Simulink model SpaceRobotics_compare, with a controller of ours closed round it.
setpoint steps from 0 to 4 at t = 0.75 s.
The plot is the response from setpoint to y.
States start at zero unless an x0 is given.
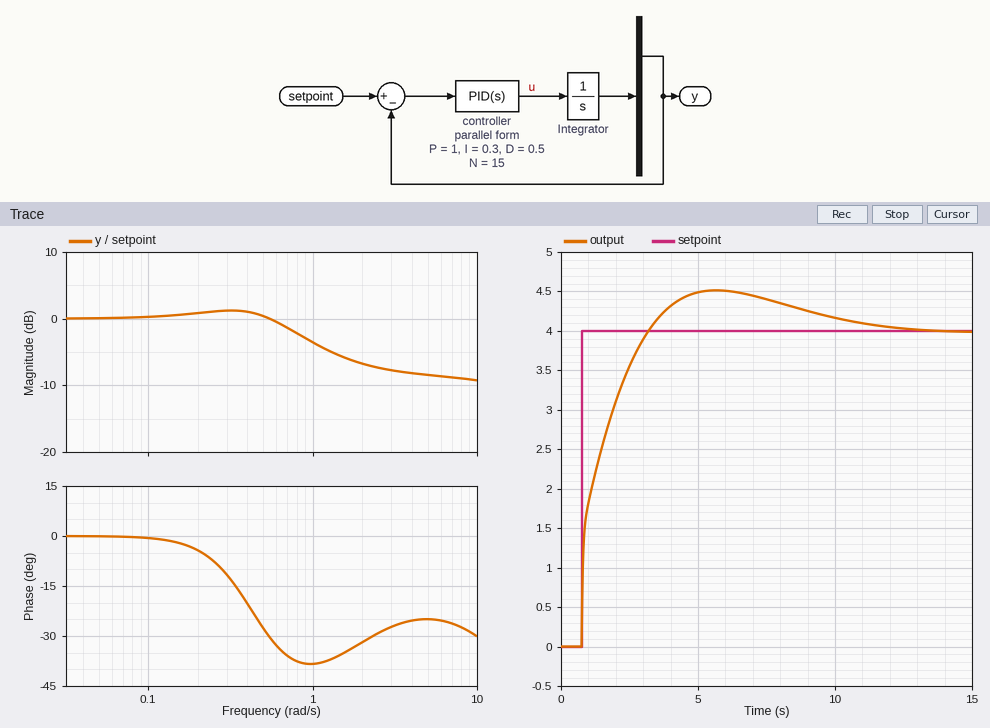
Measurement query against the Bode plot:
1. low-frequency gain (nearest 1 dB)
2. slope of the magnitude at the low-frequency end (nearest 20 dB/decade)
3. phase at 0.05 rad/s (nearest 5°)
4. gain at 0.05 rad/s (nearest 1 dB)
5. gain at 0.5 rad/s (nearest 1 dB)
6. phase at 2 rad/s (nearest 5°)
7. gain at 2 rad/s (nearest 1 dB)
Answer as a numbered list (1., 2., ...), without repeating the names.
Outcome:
1. 0 dB
2. 0 dB/decade
3. 0°
4. 0 dB
5. 0 dB
6. -30°
7. -7 dB
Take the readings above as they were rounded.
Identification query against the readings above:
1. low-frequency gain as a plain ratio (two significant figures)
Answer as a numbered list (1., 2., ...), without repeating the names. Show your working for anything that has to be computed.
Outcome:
1. 10^(0 / 20) = 1.0
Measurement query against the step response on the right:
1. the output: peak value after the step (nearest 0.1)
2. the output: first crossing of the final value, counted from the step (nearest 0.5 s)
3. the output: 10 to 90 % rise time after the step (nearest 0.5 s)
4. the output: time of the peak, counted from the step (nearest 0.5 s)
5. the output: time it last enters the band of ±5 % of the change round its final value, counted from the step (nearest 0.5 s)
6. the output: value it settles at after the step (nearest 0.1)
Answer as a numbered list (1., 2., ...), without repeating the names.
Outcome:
1. 4.5
2. 2.5 s
3. 2.0 s
4. 5.0 s
5. 9.0 s
6. 4.0
